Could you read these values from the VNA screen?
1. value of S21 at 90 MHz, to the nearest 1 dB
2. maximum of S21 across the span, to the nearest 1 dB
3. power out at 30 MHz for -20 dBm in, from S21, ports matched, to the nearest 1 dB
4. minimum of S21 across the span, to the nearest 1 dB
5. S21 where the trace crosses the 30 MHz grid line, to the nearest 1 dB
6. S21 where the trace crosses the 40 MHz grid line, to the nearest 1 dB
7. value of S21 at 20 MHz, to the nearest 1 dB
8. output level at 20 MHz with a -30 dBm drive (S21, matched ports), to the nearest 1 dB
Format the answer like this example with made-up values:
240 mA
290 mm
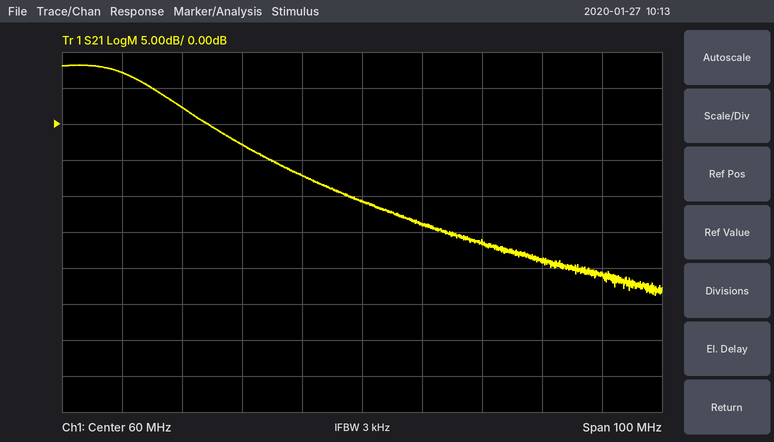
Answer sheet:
-19 dB
8 dB
-18 dBm
-24 dB
2 dB
-3 dB
7 dB
-23 dBm
